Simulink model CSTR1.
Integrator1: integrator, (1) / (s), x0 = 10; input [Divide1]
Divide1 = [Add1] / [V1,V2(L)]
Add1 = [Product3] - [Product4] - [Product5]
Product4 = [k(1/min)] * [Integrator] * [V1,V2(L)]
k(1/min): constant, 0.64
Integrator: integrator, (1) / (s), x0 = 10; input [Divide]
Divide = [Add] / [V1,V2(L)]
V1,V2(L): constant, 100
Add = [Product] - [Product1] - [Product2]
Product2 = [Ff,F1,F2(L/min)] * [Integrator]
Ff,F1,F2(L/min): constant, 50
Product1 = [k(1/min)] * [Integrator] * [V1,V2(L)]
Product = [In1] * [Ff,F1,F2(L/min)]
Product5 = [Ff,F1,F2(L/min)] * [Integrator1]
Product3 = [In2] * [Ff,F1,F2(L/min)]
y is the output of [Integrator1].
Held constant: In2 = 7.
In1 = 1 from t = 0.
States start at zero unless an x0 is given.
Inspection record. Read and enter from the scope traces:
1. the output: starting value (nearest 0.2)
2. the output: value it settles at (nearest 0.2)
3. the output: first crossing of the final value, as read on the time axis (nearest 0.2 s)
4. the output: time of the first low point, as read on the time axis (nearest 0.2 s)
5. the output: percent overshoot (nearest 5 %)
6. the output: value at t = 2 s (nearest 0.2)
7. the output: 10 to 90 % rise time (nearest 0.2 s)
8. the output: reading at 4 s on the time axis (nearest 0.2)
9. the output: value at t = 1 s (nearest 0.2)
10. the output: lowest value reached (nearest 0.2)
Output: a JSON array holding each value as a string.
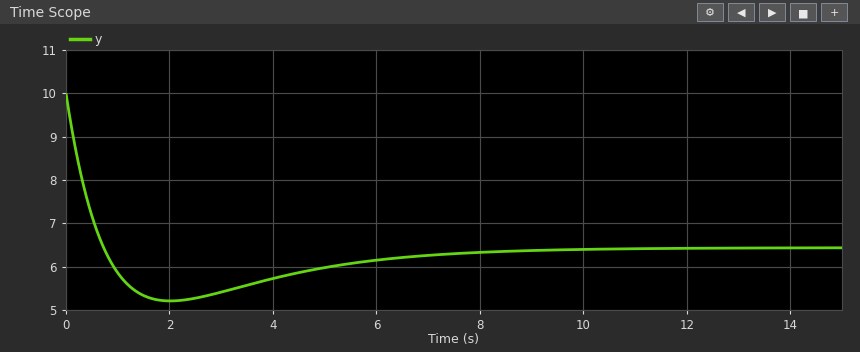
["10.0", "6.4", "0.8 s", "2.0 s", "35 %", "5.2", "0.6 s", "5.8", "5.8", "5.2"]
